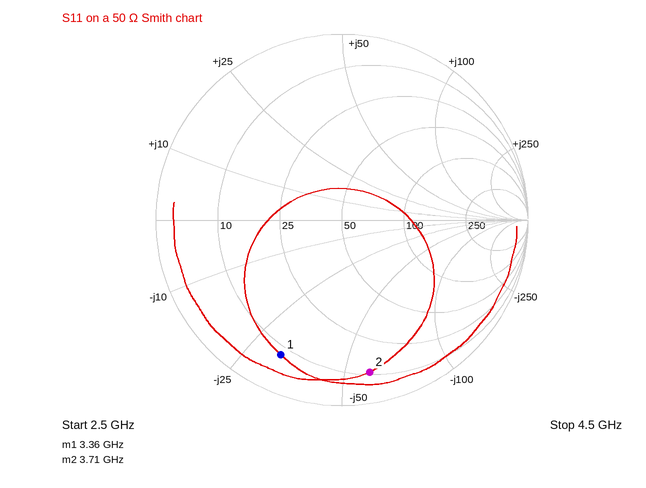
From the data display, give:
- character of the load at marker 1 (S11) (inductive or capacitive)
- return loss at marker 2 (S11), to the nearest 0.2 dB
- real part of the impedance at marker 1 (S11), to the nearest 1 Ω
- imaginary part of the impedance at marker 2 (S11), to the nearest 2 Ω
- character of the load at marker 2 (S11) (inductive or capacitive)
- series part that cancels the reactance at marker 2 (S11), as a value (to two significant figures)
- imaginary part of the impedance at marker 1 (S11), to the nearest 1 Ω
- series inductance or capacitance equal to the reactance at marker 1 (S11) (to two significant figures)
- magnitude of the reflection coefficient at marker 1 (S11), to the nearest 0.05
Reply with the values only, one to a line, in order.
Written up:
capacitive
1.6 dB
8 Ω
-58 Ω
capacitive
2.5 nH
-32 Ω
1.5 pF
0.80
